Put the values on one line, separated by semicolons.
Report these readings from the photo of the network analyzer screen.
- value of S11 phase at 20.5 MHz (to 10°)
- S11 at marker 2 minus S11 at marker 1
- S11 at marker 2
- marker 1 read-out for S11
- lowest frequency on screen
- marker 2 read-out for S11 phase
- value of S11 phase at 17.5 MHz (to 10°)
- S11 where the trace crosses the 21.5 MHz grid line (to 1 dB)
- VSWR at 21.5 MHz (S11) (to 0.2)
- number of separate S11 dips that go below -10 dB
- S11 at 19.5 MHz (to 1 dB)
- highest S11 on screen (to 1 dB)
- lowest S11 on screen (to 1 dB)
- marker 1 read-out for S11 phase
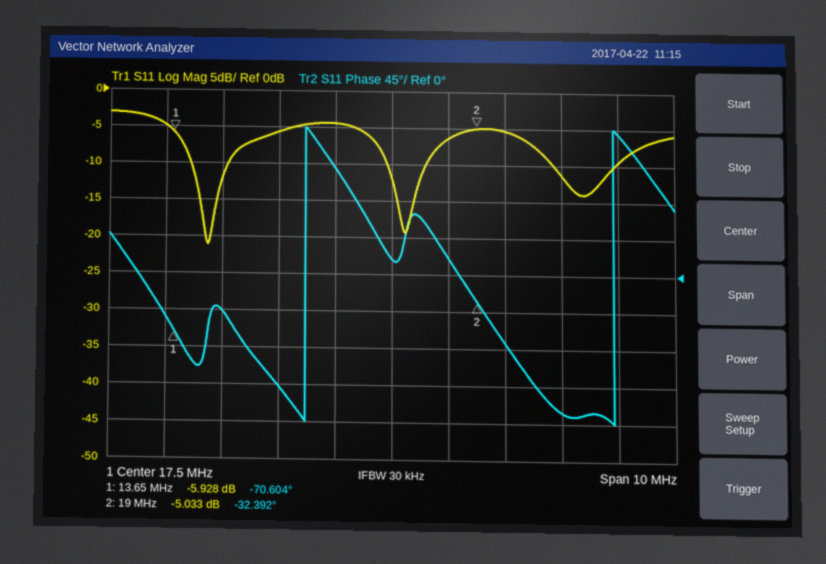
-170°; 0.895 dB; -5.033 dB; -5.928 dB; 12.5 MHz; -32.392°; 20°; -10 dB; 2.0; 3; -5 dB; -3 dB; -21 dB; -70.604°
